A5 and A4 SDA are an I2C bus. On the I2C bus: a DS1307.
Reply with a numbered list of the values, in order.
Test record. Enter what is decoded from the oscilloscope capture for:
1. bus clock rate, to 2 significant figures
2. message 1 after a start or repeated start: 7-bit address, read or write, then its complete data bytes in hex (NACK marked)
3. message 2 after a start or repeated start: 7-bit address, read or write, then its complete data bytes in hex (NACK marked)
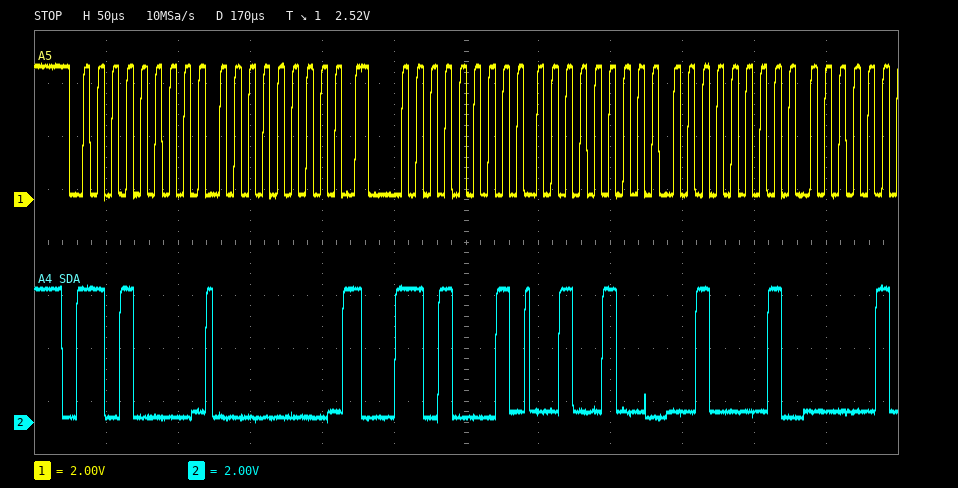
1. 100 kHz
2. 0x68 write: 00
3. 0x68 read: 24 21
